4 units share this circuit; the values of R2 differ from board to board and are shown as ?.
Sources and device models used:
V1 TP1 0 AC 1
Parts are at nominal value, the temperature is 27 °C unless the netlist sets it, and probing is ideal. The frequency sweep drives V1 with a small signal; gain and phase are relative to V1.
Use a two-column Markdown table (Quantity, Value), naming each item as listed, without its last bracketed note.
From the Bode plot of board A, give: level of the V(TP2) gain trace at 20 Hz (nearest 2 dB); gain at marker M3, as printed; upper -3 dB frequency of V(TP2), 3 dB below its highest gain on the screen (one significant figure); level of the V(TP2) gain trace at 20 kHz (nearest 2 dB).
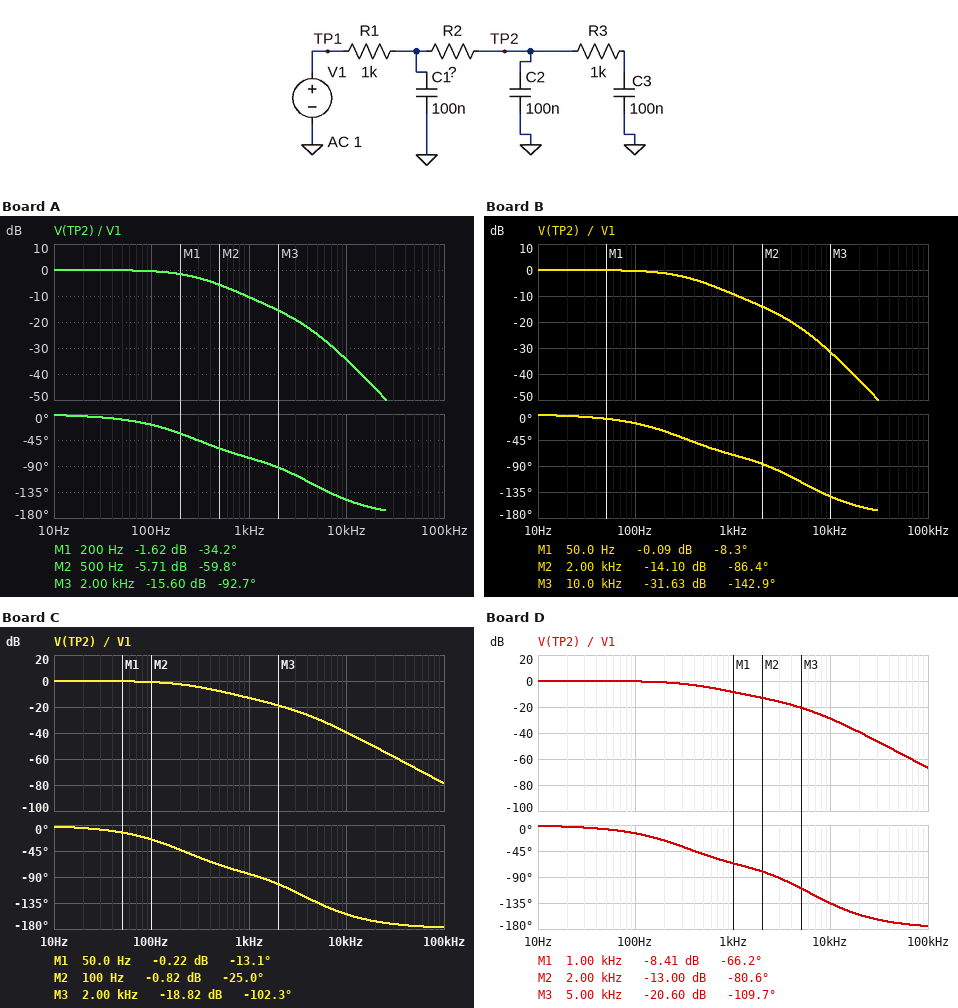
| Quantity | Value |
|---|---|
| level of the V(TP2) gain trace at 20 Hz | 0 dB |
| gain at marker M3, as printed | -15.60 dB |
| upper -3 dB frequency of V(TP2), 3 dB below its highest gain on the screen | 300 Hz |
| level of the V(TP2) gain trace at 20 kHz | -46 dB |
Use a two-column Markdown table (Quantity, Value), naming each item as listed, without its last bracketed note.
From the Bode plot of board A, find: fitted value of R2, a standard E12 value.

| Quantity | Value |
|---|---|
| fitted value of R2, a standard E12 value | 1.2 kΩ |
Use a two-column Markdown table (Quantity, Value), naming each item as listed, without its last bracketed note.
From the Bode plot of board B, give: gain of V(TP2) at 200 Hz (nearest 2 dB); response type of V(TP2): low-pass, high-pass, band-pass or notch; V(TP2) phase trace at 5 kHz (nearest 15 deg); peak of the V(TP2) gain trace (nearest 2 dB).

| Quantity | Value |
|---|---|
| gain of V(TP2) at 200 Hz | -2 dB |
| response type of V(TP2): low-pass, high-pass, band-pass or notch | low-pass |
| V(TP2) phase trace at 5 kHz | -120 deg |
| peak of the V(TP2) gain trace | 0 dB |
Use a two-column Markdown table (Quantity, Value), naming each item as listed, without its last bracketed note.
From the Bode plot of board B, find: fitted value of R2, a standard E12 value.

| Quantity | Value |
|---|---|
| fitted value of R2, a standard E12 value | 820 Ω |
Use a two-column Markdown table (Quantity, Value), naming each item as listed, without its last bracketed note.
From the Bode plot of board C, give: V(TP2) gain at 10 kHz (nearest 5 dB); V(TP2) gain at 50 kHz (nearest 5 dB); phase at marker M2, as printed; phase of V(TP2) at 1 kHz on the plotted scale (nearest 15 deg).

| Quantity | Value |
|---|---|
| V(TP2) gain at 10 kHz | -40 dB |
| V(TP2) gain at 50 kHz | -65 dB |
| phase at marker M2, as printed | -25.0 deg |
| phase of V(TP2) at 1 kHz on the plotted scale | -90 deg |
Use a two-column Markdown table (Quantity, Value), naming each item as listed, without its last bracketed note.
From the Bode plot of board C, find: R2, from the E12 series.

| Quantity | Value |
|---|---|
| R2, from the E12 series | 2.2 kΩ |
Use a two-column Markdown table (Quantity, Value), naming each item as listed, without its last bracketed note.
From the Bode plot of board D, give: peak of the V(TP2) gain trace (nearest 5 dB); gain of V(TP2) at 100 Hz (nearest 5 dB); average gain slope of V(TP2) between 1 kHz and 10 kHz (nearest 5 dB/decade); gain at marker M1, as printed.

| Quantity | Value |
|---|---|
| peak of the V(TP2) gain trace | 0 dB |
| gain of V(TP2) at 100 Hz | 0 dB |
| average gain slope of V(TP2) between 1 kHz and 10 kHz | -20 dB/decade |
| gain at marker M1, as printed | -8.41 dB |
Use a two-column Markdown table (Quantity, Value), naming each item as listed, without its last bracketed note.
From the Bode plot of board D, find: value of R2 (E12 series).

| Quantity | Value |
|---|---|
| value of R2 | 560 Ω |
